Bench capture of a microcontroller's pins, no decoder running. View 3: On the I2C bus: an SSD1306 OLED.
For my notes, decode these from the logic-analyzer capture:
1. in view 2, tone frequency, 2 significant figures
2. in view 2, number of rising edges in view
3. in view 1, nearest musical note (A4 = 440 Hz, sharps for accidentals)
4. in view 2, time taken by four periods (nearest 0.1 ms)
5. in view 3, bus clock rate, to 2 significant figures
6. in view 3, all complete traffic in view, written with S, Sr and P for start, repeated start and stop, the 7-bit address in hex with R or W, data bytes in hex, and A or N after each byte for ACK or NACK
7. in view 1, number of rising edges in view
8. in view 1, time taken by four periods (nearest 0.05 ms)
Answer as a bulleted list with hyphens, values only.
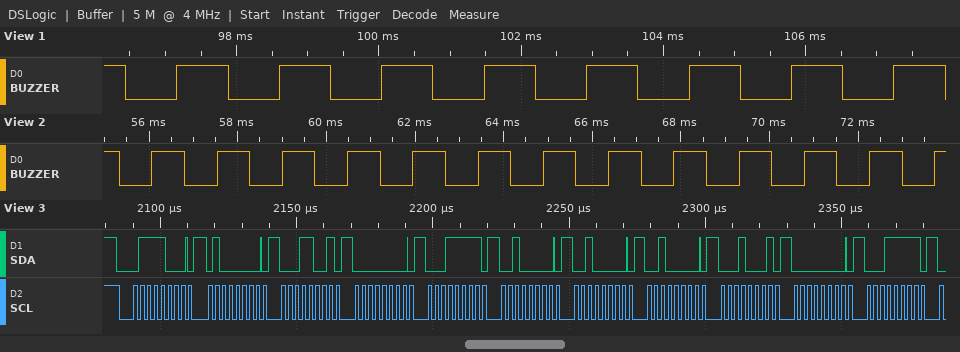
- 680 Hz
- 13
- F5
- 5.9 ms
- 400 kHz
- S 3CW A 40 A 19 A 00 A 1F A 20 A 20 A 20 A 11 A 00 A 1F A
- 8
- 5.75 ms
